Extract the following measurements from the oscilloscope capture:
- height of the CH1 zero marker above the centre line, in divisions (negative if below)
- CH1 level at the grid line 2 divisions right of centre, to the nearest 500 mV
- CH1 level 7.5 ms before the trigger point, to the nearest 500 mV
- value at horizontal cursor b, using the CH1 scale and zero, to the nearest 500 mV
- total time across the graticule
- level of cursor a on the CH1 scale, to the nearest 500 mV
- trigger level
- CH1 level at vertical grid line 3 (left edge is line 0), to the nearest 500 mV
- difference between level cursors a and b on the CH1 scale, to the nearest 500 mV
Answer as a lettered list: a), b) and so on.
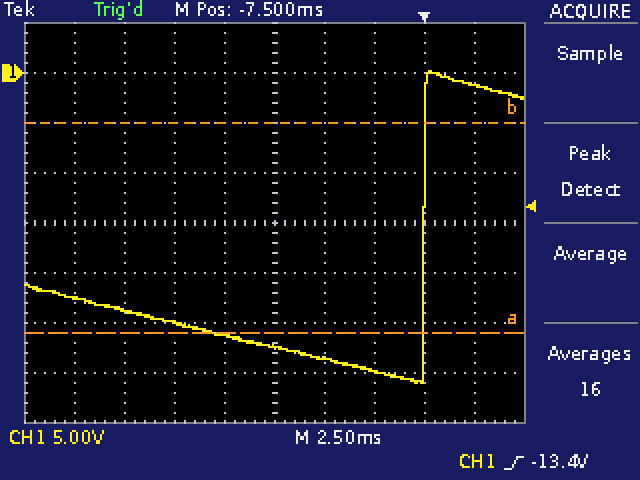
a) +3.0 div
b) -30.0 V
c) -27.5 V
d) -5.0 V
e) 25 ms
f) -26.0 V
g) -13.4 V
h) -25.0 V
i) 21.0 V
